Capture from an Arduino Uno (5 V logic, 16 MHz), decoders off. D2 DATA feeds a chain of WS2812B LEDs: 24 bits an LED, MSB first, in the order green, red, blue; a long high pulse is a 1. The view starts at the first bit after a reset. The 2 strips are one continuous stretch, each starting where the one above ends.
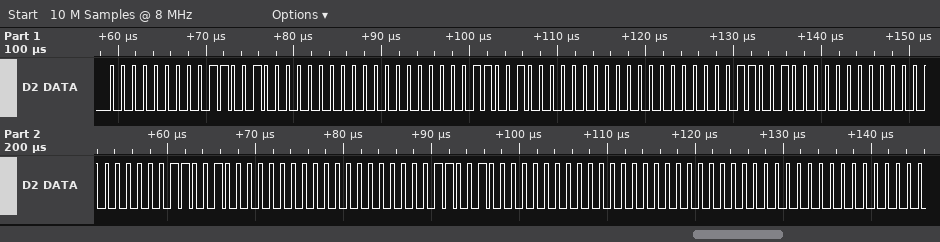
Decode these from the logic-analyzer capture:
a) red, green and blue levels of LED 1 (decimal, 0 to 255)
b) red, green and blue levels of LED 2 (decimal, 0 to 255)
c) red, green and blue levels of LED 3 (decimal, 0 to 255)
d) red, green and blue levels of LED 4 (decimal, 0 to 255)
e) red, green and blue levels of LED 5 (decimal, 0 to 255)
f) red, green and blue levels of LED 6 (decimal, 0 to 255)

100, 0, 0
100, 0, 0
100, 0, 0
100, 0, 0
100, 0, 0
0, 0, 0
